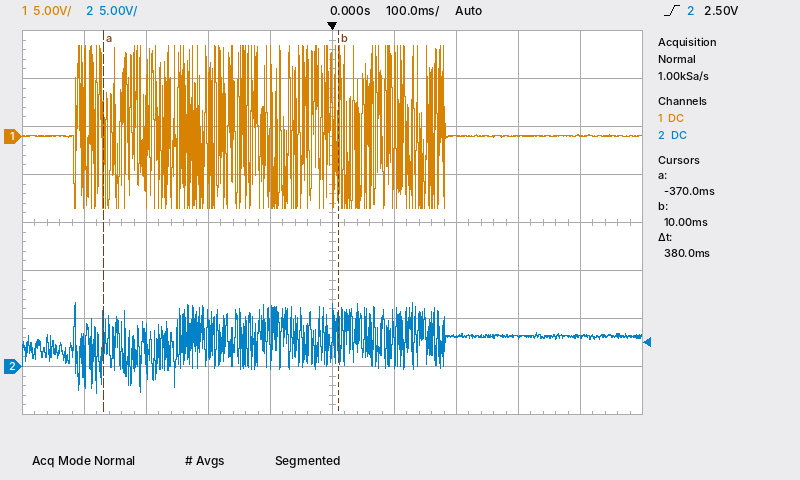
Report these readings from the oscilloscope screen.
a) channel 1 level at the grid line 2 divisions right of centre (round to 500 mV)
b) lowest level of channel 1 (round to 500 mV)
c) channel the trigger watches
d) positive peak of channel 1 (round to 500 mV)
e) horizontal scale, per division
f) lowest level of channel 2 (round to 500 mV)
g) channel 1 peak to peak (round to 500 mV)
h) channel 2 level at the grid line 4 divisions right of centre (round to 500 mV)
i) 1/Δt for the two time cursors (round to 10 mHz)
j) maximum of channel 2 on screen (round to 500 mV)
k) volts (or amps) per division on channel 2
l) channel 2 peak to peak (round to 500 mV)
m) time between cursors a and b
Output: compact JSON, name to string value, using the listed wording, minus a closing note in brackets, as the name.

{"channel 1 level at the grid line 2 divisions right of centre": "0.0 V", "lowest level of channel 1": "-7.5 V", "channel the trigger watches": "channel 2", "positive peak of channel 1": "9.5 V", "horizontal scale, per division": "100 ms", "lowest level of channel 2": "-3.0 V", "channel 1 peak to peak": "17.0 V", "channel 2 level at the grid line 4 divisions right of centre": "3.0 V", "1/Δt for the two time cursors": "2.63 Hz", "maximum of channel 2 on screen": "6.5 V", "volts (or amps) per division on channel 2": "5 V", "channel 2 peak to peak": "9.5 V", "time between cursors a and b": "380 ms"}
